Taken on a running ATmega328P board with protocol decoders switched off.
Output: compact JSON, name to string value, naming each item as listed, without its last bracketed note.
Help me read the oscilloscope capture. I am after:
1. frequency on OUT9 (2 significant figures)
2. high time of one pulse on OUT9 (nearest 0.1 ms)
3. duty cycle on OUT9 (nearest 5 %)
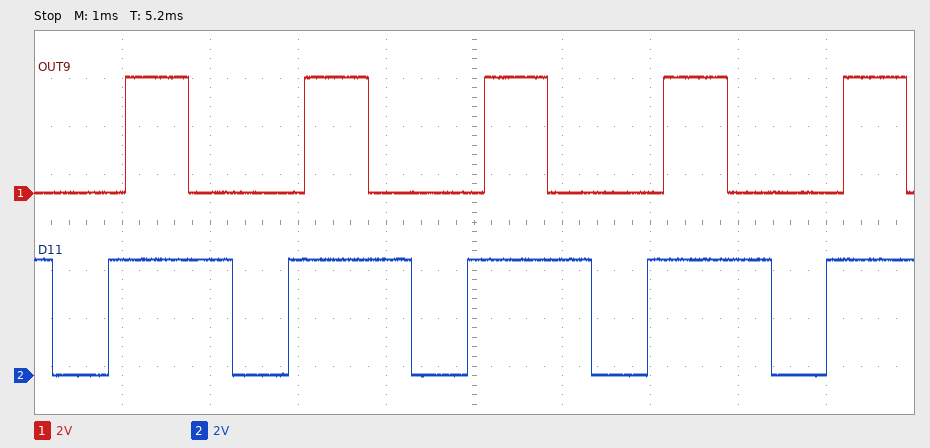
{"frequency on OUT9": "490 Hz", "high time of one pulse on OUT9": "0.7 ms", "duty cycle on OUT9": "35 %"}
